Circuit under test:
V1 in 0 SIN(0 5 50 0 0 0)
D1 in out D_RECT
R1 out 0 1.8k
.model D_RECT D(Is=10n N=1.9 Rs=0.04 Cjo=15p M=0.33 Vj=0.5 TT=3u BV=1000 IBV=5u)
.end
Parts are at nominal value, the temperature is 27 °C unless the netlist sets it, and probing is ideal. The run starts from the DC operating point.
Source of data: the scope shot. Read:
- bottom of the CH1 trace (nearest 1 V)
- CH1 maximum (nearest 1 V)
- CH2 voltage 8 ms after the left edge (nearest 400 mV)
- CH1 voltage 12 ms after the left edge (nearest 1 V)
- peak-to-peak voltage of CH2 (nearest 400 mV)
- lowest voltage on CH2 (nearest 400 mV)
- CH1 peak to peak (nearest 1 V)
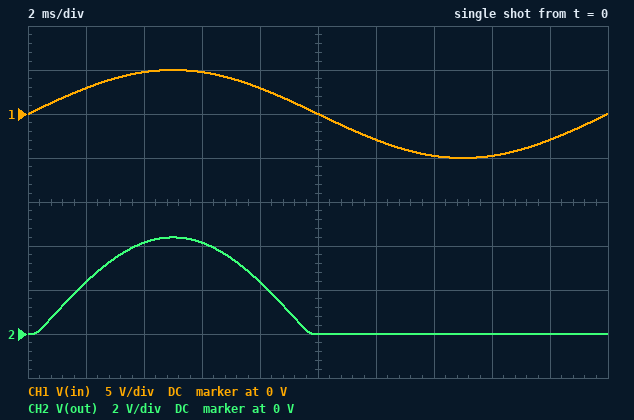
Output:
-5 V
5 V
2.4 V
-3 V
4.4 V
0 V
10 V
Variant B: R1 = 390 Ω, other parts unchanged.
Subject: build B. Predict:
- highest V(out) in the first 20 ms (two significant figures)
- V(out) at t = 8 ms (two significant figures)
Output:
4.3 V
2.3 V
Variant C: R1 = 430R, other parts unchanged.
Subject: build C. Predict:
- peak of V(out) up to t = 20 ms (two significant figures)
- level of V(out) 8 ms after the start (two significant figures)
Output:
4.3 V
2.3 V
